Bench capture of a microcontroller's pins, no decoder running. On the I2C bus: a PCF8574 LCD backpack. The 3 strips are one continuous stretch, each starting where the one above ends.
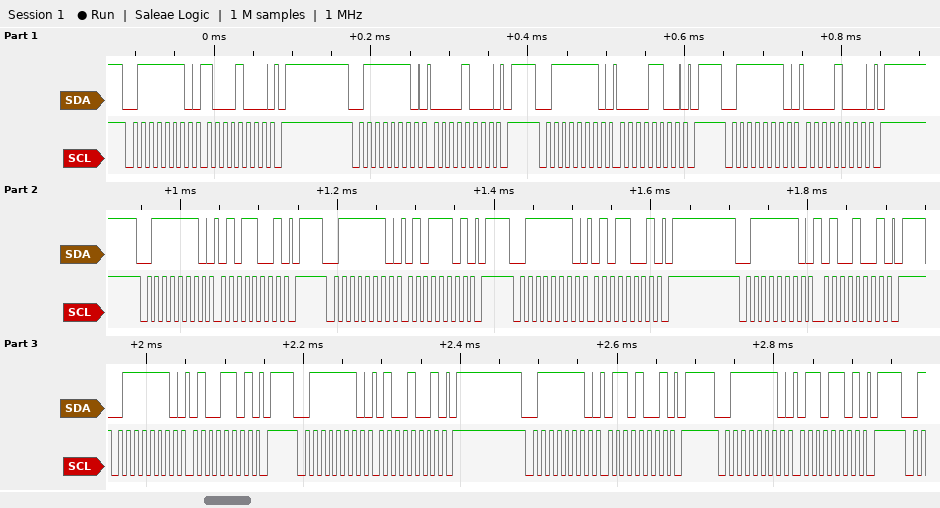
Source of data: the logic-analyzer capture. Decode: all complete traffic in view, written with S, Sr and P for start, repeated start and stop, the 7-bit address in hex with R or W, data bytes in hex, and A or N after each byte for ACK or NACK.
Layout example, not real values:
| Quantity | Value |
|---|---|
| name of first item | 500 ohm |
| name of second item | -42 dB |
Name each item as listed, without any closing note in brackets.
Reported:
| Quantity | Value |
|---|---|
| all complete traffic in view, written with S, Sr and P for start, repeated start and stop, the 7-bit address in hex with R or W, data bytes in hex, and A or N after each byte for ACK or NACK | S 3FW A 88 A P S 3FW A 08 A P S 3FW A 0C A P S 3FW A 08 A P S 3FW A 59 A P S 3FW A 5D A P S 3FW A 59 A P S 3FW A 49 A P S 3FW A 4D A P S 3FW A 49 A P S 3FW A 69 A P S 3FW A 6D A P |
